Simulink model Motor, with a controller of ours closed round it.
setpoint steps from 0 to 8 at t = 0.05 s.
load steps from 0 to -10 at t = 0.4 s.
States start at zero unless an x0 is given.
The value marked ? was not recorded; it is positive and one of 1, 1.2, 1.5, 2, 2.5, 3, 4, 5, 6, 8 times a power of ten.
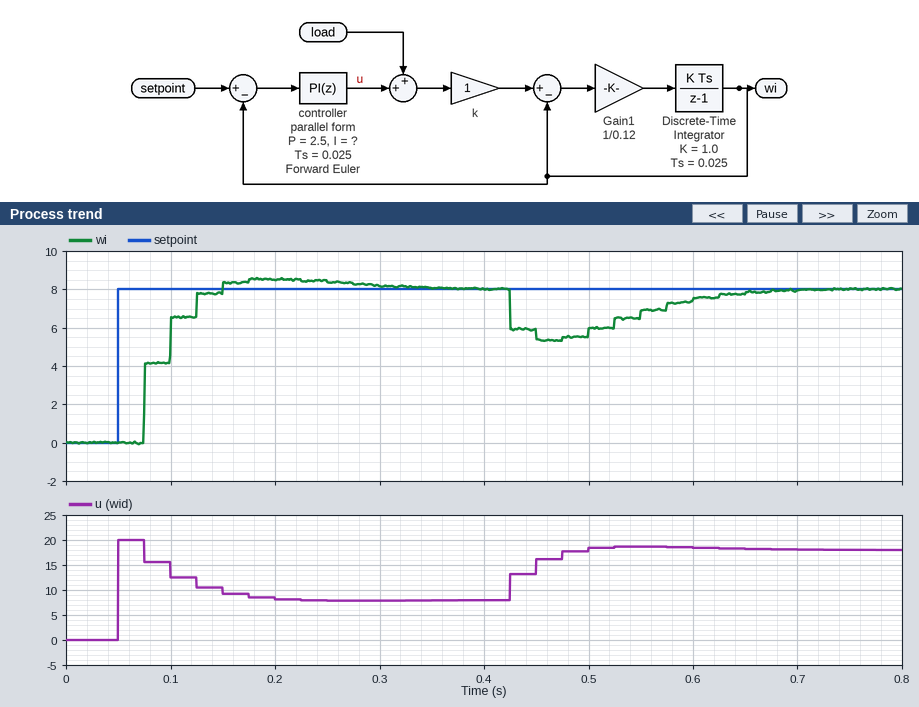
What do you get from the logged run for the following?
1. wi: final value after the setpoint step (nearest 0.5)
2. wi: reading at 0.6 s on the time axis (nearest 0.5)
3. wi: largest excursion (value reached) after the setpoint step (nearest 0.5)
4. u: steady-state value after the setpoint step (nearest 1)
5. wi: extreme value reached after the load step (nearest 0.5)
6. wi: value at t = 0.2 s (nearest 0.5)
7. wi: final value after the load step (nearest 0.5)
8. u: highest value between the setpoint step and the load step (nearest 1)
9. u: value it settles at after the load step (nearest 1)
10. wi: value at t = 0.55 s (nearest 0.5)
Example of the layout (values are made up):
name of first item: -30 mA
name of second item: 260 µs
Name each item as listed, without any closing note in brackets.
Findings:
wi: final value after the setpoint step: 8.0
wi: reading at 0.6 s on the time axis: 7.5
wi: largest excursion (value reached) after the setpoint step: 8.5
u: steady-state value after the setpoint step: 8
wi: extreme value reached after the load step: 5.5
wi: value at t = 0.2 s: 8.5
wi: final value after the load step: 8.0
u: highest value between the setpoint step and the load step: 20
u: value it settles at after the load step: 18
wi: value at t = 0.55 s: 7.0
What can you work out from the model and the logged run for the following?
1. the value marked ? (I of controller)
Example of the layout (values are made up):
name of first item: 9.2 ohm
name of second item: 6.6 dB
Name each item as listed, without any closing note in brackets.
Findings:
the value marked ?: 30
